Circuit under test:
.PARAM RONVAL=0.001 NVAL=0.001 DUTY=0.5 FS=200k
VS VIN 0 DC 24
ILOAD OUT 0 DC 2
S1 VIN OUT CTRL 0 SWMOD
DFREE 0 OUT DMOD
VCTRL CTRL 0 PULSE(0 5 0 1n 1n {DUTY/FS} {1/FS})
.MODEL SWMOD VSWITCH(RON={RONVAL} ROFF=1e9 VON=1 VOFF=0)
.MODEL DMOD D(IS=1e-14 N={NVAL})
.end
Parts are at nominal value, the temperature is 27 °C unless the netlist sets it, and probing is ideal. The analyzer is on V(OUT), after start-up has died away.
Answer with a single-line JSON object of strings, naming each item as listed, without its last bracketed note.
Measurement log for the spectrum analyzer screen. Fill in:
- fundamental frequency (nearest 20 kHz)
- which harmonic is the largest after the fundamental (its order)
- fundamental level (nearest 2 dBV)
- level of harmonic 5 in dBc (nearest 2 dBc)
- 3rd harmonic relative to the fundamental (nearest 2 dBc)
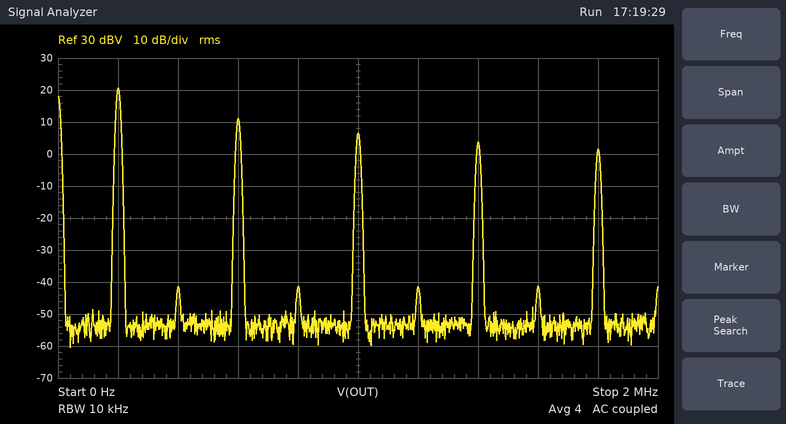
{"fundamental frequency": "200 kHz", "which harmonic is the largest after the fundamental": "3", "fundamental level": "20 dBV", "level of harmonic 5 in dBc": "-14 dBc", "3rd harmonic relative to the fundamental": "-10 dBc"}
